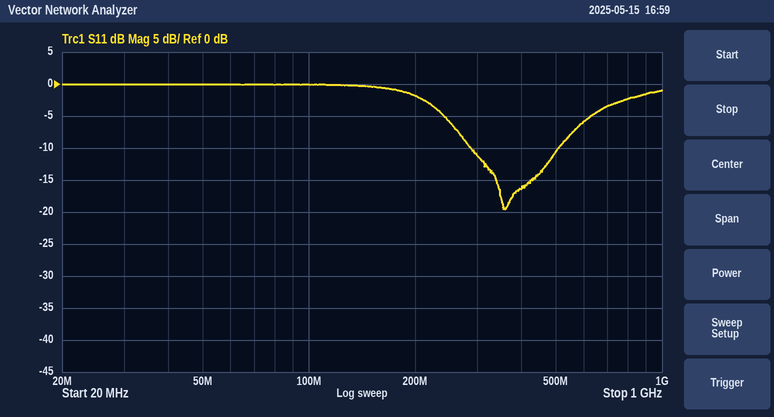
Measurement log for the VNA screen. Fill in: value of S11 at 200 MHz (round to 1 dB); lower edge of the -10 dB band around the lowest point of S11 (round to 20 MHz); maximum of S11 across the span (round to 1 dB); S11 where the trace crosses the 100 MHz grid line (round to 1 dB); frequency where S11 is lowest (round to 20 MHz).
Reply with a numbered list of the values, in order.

1. -2 dB
2. 280 MHz
3. 0 dB
4. 0 dB
5. 360 MHz
